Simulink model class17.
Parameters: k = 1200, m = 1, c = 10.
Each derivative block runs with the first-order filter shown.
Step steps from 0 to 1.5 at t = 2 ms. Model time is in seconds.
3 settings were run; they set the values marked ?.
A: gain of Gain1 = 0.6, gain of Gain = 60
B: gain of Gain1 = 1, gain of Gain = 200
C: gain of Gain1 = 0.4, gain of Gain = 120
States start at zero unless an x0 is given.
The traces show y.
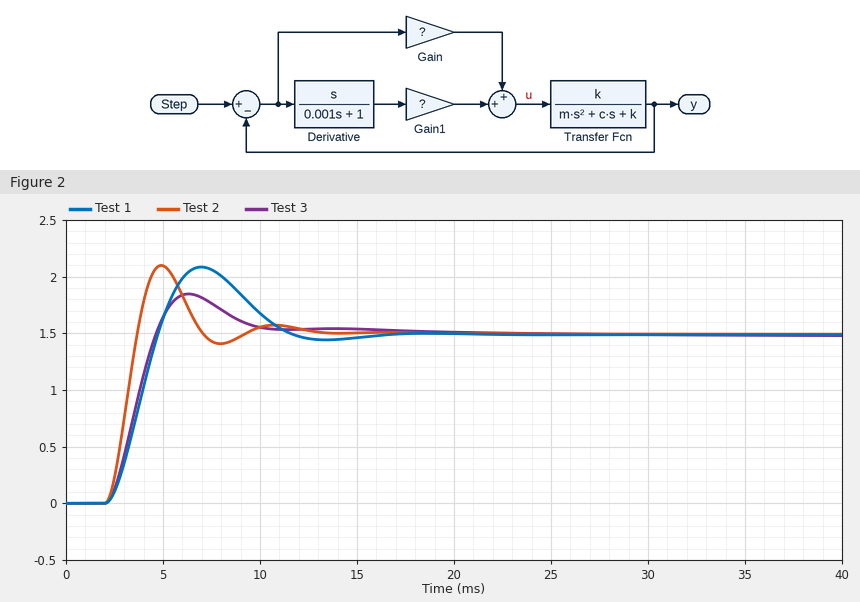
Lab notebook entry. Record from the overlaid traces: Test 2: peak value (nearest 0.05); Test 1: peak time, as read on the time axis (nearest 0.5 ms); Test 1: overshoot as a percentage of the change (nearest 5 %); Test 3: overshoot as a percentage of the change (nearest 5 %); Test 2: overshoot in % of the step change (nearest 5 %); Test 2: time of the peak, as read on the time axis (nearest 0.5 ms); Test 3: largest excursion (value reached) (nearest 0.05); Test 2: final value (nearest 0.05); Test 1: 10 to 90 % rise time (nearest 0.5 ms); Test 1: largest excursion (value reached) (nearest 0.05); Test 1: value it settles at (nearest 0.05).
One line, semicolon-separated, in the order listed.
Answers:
2.10; 7.0 ms; 40 %; 25 %; 40 %; 5.0 ms; 1.85; 1.50; 2.0 ms; 2.10; 1.50
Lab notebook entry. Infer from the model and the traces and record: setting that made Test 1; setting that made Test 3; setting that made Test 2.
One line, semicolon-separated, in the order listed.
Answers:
C; A; B
